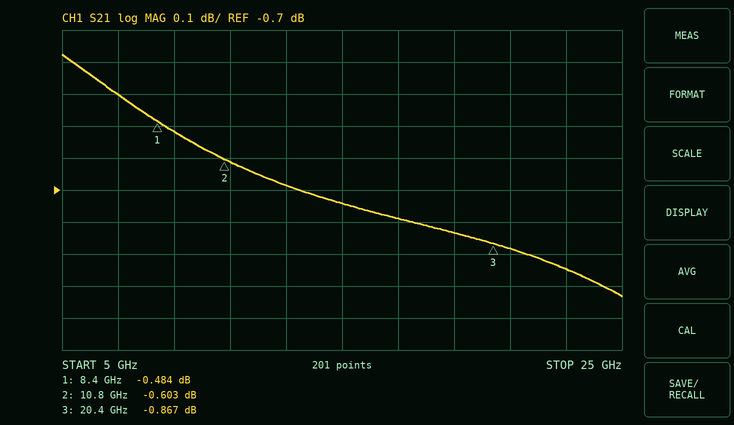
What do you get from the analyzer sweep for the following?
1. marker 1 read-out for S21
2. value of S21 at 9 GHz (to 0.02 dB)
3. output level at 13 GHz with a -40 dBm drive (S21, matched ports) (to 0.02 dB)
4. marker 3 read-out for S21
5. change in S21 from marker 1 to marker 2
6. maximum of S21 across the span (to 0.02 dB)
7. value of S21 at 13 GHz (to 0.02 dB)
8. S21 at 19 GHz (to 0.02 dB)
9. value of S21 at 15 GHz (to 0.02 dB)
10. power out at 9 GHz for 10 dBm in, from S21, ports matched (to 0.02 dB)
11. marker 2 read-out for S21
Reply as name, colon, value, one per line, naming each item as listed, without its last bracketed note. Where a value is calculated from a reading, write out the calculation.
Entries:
marker 1 read-out for S21: -0.484 dB
value of S21 at 9 GHz: -0.52 dB
output level at 13 GHz with a -40 dBm drive (S21, matched ports): -40 dBm + (-0.68 dB) = -40.68 dBm
marker 3 read-out for S21: -0.867 dB
change in S21 from marker 1 to marker 2: -0.603 − (-0.484) = -0.119 dB
maximum of S21 across the span: -0.28 dB
value of S21 at 13 GHz: -0.68 dB
S21 at 19 GHz: -0.84 dB
value of S21 at 15 GHz: -0.74 dB
power out at 9 GHz for 10 dBm in, from S21, ports matched: 10 dBm + (-0.52 dB) = 9.48 dBm
marker 2 read-out for S21: -0.603 dB
